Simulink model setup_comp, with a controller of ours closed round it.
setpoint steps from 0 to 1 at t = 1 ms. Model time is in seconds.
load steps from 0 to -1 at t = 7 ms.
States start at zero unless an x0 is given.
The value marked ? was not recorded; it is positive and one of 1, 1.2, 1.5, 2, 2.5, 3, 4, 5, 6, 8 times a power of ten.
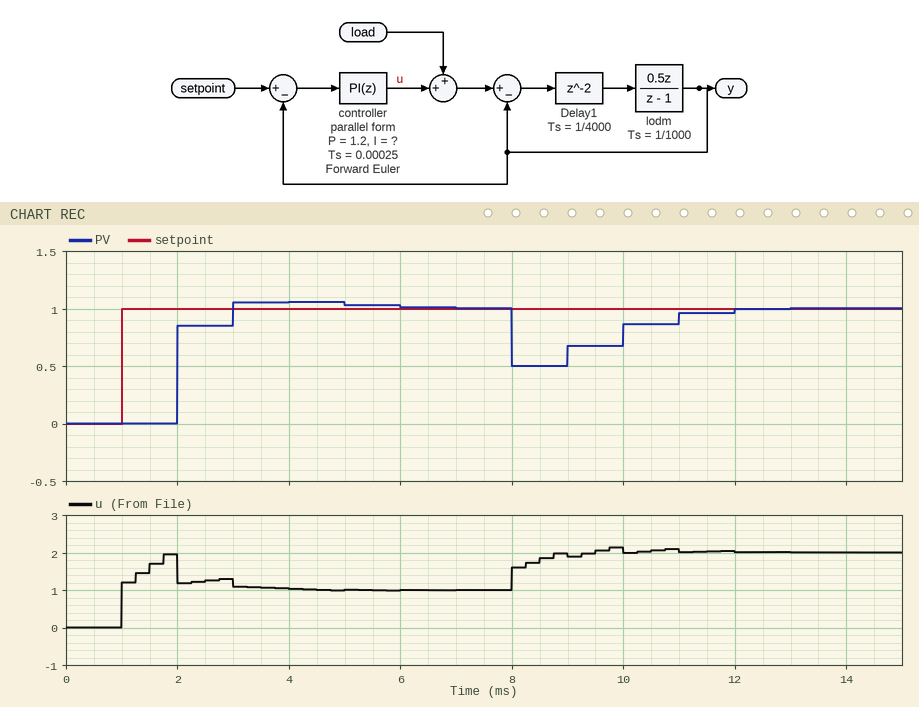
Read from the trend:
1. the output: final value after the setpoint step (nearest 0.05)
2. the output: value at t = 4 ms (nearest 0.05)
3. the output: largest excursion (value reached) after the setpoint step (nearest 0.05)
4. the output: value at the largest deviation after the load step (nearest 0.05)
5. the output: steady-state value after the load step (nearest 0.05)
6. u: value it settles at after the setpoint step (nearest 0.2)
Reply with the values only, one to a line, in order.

1.00
1.05
1.05
0.50
1.00
1.0
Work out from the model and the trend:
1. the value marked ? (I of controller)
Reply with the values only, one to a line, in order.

1000
